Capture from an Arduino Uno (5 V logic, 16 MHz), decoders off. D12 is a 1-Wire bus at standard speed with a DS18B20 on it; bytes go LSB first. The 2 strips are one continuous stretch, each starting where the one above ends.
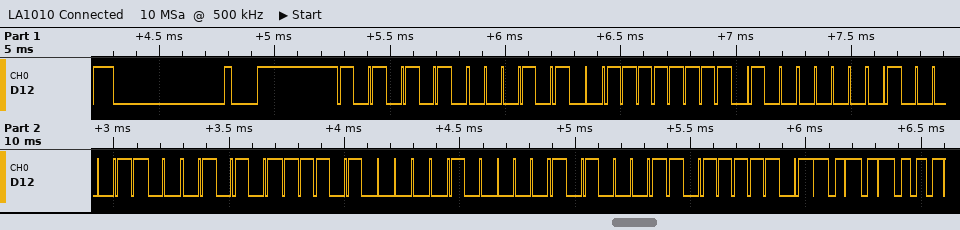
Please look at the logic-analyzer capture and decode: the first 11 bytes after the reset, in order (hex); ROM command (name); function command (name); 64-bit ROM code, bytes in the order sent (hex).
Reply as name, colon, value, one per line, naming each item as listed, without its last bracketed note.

the first 11 bytes after the reset, in order: 55 28 FF 02 C2 A8 17 04 C5 BE 15
ROM command: Match ROM
function command: Read Scratchpad
64-bit ROM code, bytes in the order sent: 28 FF 02 C2 A8 17 04 C5
